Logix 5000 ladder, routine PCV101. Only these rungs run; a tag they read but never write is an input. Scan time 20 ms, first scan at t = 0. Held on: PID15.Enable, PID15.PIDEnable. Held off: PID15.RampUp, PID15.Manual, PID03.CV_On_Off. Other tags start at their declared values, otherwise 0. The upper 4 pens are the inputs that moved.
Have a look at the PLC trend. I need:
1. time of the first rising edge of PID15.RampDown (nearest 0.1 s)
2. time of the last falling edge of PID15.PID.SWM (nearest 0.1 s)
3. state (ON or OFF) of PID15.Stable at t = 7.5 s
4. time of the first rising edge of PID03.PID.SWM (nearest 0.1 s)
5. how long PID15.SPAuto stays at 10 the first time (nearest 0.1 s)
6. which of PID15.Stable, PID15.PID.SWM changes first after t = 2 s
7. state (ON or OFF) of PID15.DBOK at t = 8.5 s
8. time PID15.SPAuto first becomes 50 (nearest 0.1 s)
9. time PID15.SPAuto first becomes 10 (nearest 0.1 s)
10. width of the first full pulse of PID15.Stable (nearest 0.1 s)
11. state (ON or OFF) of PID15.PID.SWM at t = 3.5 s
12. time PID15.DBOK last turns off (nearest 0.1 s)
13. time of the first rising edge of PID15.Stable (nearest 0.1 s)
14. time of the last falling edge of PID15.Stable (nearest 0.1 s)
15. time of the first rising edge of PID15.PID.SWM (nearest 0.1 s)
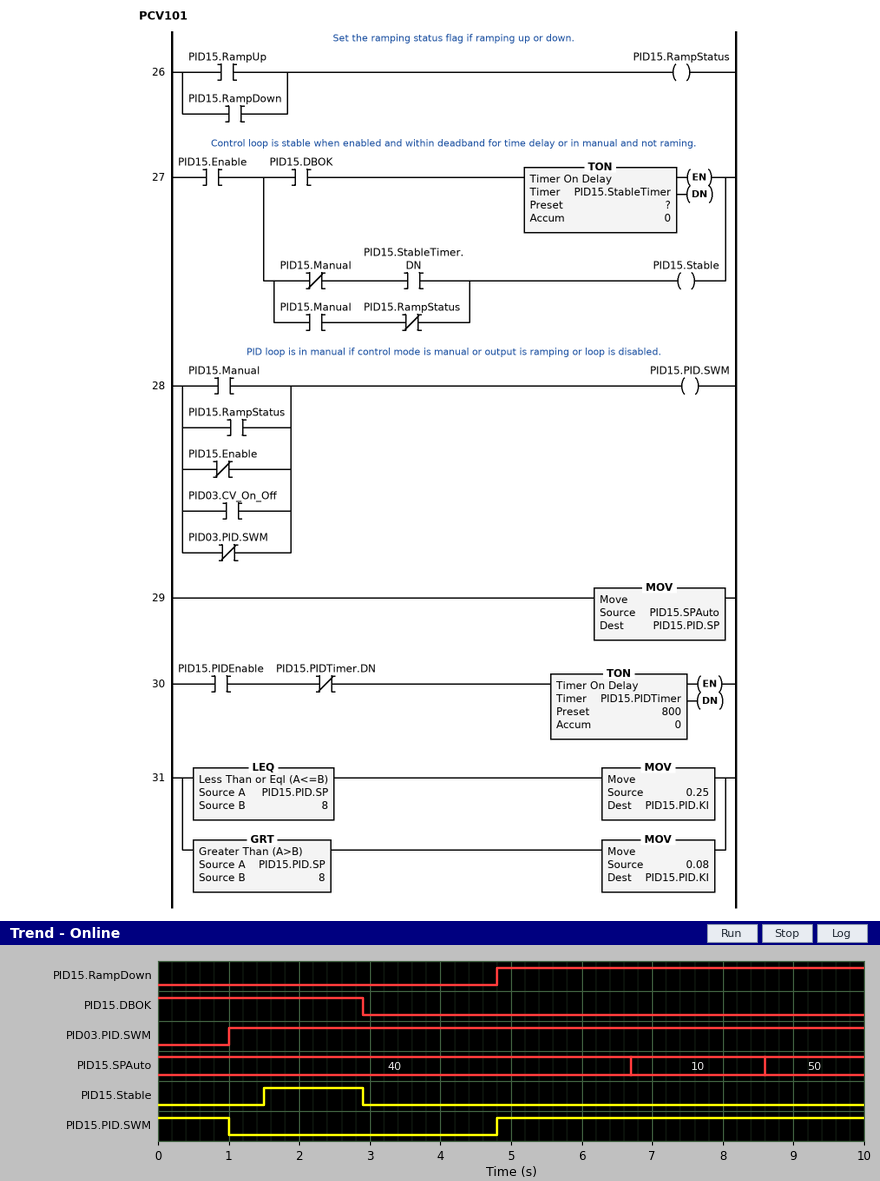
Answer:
4.8 s
1.0 s
OFF
1.0 s
1.9 s
PID15.Stable
OFF
8.6 s
6.7 s
1.4 s
OFF
2.9 s
1.5 s
2.9 s
4.8 s
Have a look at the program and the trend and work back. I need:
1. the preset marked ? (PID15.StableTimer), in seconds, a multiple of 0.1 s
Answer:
1.5 s
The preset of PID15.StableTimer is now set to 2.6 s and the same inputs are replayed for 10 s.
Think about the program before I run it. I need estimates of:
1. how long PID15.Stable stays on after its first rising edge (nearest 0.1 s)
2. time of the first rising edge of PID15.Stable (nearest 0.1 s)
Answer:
0.3 s
2.6 s
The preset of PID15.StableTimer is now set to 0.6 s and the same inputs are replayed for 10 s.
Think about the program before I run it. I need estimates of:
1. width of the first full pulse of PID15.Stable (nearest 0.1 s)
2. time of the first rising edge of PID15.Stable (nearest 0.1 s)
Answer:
2.3 s
0.6 s
